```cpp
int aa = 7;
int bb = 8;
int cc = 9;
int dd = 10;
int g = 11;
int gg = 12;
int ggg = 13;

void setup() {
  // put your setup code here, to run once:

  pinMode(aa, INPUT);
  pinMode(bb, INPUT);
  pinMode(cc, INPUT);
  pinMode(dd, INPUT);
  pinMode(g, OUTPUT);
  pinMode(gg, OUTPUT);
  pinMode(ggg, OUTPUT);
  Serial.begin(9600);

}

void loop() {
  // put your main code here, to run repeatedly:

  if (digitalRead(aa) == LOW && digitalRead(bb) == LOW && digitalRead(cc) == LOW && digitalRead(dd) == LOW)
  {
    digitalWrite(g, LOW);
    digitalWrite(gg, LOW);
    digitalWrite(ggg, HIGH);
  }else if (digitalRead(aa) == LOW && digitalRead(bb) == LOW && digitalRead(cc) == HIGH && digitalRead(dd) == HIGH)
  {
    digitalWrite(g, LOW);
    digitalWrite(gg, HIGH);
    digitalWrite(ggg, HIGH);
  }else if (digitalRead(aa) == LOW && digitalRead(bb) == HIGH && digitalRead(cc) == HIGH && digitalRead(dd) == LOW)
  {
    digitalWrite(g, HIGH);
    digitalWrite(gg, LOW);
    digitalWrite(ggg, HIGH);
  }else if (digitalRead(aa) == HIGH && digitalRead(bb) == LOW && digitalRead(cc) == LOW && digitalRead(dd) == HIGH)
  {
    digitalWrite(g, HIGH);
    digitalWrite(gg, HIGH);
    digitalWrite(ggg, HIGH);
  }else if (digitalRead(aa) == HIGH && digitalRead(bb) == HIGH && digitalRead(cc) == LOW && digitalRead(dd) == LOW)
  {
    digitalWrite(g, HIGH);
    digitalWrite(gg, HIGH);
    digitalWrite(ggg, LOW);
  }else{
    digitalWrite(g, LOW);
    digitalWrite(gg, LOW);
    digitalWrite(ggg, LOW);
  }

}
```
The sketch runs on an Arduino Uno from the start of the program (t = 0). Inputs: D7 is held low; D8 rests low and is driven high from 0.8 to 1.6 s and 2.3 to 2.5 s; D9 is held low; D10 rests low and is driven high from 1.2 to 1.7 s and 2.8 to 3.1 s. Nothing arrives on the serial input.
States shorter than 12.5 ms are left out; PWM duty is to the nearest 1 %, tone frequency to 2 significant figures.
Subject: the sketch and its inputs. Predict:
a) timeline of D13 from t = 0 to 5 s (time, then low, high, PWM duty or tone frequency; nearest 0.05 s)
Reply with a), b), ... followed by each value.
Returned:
a) 0 s high; 0.8 s low; 1.7 s high; 2.3 s low; 2.5 s high; 2.8 s low; 3.1 s high
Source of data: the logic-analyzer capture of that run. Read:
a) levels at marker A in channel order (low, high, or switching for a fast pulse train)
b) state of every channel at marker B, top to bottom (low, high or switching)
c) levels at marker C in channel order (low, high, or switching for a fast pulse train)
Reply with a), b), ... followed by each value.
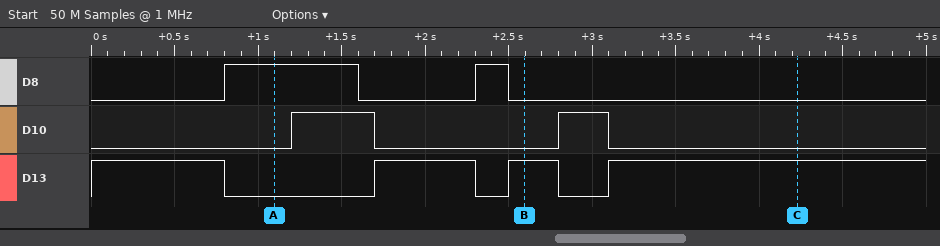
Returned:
a) D8 high, D10 low, D13 low
b) D8 low, D10 low, D13 high
c) D8 low, D10 low, D13 high
